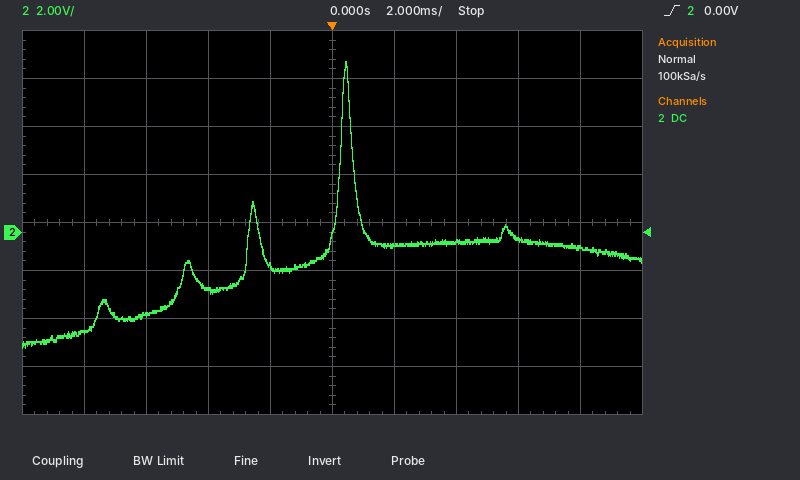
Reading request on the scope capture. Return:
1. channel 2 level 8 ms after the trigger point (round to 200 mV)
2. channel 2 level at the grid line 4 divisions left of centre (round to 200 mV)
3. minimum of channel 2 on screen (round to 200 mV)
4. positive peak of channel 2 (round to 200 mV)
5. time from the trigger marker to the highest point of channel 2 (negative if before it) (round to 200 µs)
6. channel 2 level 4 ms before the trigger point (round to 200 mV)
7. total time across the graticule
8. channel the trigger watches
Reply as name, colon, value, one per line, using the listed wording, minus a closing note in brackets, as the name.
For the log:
channel 2 level 8 ms after the trigger point: -600 mV
channel 2 level at the grid line 4 divisions left of centre: -4.2 V
minimum of channel 2 on screen: -4.8 V
positive peak of channel 2: 7.2 V
time from the trigger marker to the highest point of channel 2 (negative if before it): +400 µs
channel 2 level 4 ms before the trigger point: -2.4 V
total time across the graticule: 20 ms
channel the trigger watches: channel 2
